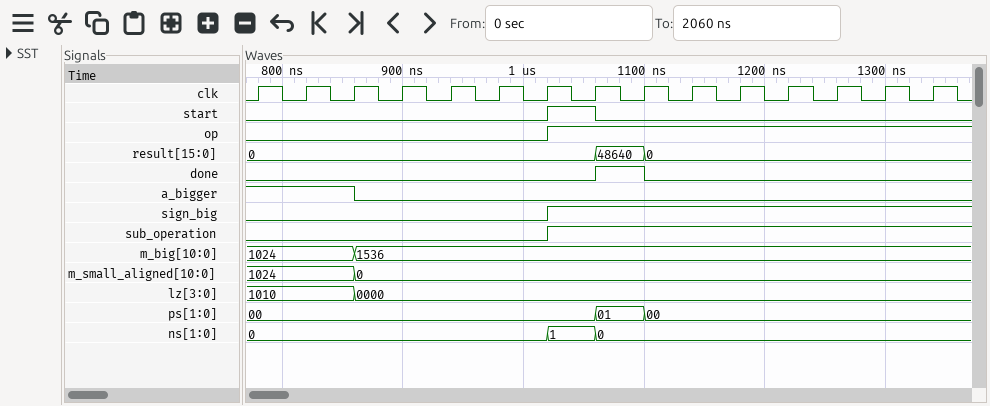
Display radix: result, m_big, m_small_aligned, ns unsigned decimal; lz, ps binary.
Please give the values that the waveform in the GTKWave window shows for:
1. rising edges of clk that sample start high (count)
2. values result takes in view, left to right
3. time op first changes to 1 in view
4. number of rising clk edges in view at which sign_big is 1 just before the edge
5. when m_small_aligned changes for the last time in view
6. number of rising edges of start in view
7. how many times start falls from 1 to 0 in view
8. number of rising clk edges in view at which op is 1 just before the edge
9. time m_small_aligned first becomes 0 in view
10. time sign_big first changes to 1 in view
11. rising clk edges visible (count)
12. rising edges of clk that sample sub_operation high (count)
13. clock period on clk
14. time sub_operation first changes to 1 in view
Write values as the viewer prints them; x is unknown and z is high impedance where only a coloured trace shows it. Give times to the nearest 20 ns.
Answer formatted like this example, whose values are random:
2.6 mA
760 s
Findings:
1
0, 48640, 0
1020 ns
8
860 ns
1
1
8
860 ns
1020 ns
15
8
40 ns
1020 ns
